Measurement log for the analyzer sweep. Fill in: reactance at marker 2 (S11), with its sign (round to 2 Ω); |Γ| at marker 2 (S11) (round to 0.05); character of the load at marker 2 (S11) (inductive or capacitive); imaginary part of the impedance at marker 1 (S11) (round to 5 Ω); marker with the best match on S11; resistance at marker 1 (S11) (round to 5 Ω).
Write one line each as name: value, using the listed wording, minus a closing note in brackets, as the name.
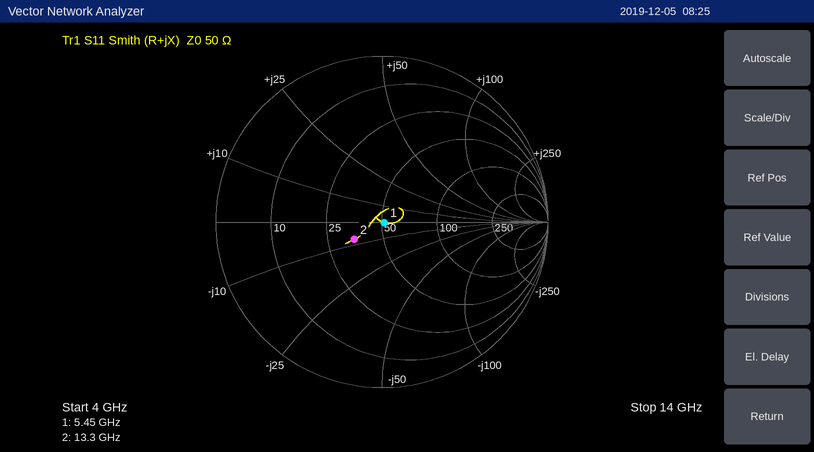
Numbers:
reactance at marker 2 (S11), with its sign: -8 Ω
|Γ| at marker 2 (S11): 0.20
character of the load at marker 2 (S11): capacitive
imaginary part of the impedance at marker 1 (S11): 0 Ω
marker with the best match on S11: marker 1
resistance at marker 1 (S11): 50 Ω
